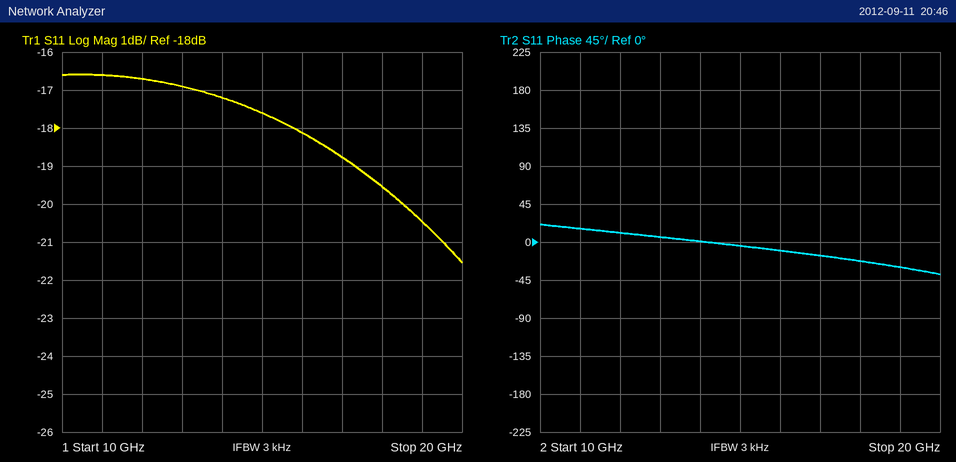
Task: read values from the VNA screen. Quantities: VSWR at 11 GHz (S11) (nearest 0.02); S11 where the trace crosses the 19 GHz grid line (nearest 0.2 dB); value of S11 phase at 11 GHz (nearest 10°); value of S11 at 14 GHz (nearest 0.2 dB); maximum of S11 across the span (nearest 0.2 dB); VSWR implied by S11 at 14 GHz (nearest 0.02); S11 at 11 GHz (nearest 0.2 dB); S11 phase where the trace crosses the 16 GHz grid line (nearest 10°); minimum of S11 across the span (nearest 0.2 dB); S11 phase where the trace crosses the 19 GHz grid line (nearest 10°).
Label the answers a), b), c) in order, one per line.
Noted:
a) 1.34
b) -20.4 dB
c) 20°
d) -17.2 dB
e) -16.6 dB
f) 1.32
g) -16.6 dB
h) -10°
i) -21.6 dB
j) -30°
